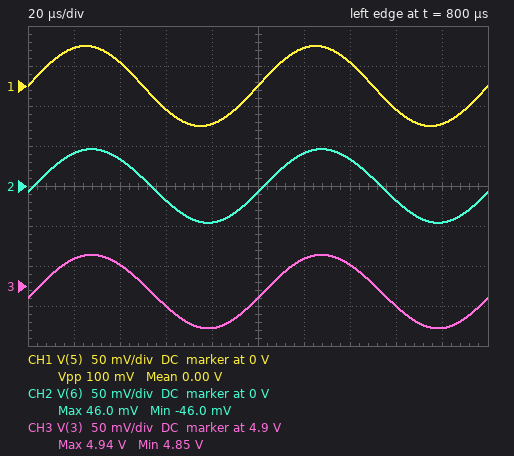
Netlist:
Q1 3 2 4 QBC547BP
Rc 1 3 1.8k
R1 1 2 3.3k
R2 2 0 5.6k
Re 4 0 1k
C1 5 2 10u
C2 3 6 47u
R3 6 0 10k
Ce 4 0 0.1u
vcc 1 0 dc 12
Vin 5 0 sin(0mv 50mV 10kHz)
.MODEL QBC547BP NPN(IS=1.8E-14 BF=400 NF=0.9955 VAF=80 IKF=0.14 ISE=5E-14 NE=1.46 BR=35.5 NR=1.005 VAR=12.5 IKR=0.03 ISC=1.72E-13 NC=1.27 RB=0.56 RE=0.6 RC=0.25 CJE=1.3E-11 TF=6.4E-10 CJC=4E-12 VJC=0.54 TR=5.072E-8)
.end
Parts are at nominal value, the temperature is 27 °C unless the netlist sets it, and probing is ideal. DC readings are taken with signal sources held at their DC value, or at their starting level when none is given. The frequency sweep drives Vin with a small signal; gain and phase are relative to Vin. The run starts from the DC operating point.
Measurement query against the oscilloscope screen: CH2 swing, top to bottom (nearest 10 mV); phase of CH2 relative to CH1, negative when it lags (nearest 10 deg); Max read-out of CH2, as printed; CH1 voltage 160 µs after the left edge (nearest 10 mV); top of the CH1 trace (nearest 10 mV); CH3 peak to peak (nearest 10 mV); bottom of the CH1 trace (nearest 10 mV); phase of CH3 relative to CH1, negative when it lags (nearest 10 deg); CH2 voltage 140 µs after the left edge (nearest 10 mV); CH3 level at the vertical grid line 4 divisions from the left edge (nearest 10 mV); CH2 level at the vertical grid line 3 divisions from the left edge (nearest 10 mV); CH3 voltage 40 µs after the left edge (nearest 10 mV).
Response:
90 mV
-10 deg
46.0 mV
-30 mV
50 mV
90 mV
-50 mV
-10 deg
30 mV
4.85 V
-20 mV
4.93 V
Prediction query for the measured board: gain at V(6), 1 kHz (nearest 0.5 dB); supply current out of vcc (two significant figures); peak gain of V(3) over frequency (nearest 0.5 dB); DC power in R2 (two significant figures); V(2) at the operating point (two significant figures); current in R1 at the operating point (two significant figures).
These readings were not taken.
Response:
-0.5 dB
5.9 mA
-0.5 dB
5.6 mW
5.6 V
1.9 mA
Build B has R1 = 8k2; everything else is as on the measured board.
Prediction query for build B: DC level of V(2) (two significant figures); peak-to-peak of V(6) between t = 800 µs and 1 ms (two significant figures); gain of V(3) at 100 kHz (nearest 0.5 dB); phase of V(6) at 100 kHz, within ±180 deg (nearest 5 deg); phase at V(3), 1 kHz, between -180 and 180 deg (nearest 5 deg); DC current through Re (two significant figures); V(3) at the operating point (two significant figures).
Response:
4.8 V
840 mV
38.5 dB
-115 deg
-150 deg
4.1 mA
4.6 V
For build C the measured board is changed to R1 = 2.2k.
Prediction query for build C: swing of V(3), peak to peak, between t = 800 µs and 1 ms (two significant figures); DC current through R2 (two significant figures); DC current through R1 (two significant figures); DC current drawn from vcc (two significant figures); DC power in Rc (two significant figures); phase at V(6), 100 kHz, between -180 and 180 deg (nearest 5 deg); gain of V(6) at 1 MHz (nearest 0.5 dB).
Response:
95 mV
1.1 mA
2.7 mA
6.4 mA
25 mW
-30 deg
-7.5 dB
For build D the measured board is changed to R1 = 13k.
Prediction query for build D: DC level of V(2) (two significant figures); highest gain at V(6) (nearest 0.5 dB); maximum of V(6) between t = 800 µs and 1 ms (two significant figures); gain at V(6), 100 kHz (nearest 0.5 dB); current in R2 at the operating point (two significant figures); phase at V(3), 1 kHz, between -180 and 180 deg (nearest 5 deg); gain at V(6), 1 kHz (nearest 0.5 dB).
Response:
3.6 V
43.5 dB
480 mV
38.0 dB
640 µA
-150 deg
5.0 dB
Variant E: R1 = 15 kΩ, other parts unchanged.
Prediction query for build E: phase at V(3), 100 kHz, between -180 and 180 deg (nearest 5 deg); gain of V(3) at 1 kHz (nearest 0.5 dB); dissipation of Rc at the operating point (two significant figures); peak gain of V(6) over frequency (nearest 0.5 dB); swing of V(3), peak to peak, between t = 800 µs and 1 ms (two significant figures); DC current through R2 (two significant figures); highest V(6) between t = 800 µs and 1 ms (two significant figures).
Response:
-125 deg
5.0 dB
12 mW
42.5 dB
950 mV
580 µA
480 mV
